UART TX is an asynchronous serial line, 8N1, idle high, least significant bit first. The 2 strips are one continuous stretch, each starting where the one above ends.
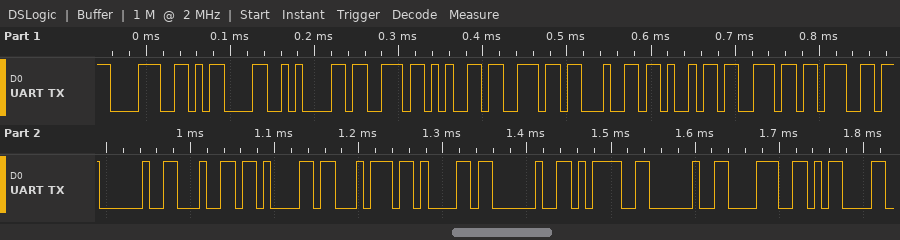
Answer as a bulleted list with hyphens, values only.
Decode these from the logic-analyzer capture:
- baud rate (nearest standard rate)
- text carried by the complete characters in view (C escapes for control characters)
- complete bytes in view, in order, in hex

- 115200 baud
- "8\r\nsending data = 8\r"
- 38 0D 0A 73 65 6E 64 69 6E 67 20 64 61 74 61 20 3D 20 38 0D
